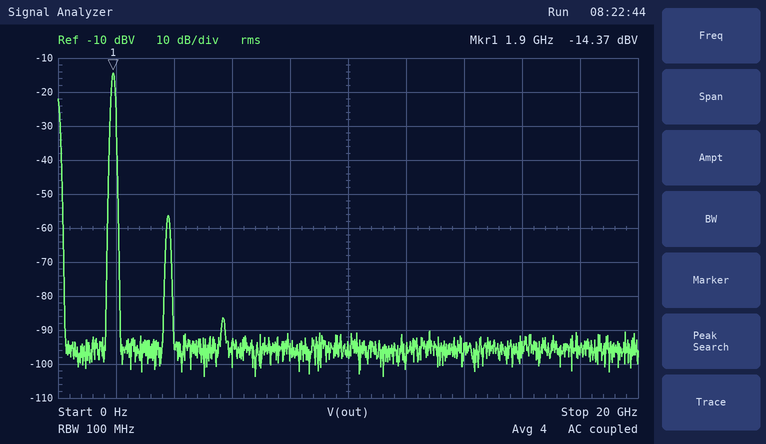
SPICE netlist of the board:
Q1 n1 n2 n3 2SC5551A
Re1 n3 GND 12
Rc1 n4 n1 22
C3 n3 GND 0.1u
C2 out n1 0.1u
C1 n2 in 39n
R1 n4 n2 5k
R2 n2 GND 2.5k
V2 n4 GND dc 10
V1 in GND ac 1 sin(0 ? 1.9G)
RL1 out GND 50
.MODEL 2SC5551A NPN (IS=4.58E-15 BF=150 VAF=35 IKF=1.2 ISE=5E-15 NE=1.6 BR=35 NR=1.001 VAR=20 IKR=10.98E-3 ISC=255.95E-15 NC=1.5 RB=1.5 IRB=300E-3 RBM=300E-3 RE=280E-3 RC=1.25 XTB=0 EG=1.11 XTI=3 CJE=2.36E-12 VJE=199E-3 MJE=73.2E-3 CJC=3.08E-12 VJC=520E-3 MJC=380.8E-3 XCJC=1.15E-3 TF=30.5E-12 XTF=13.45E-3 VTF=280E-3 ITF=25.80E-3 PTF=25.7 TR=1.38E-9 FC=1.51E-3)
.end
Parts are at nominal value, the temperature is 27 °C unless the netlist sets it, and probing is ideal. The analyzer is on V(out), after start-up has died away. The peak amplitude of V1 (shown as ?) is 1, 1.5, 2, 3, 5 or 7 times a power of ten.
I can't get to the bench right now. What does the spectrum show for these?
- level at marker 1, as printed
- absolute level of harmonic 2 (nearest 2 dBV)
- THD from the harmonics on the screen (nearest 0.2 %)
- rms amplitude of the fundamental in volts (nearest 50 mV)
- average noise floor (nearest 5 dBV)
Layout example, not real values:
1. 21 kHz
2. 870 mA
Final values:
1. -14.37 dBV
2. -56 dBV
3. 0.8 %
4. 200 mV
5. -95 dBV
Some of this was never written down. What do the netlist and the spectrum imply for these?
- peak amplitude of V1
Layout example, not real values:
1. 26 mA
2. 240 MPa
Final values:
1. 15 mV
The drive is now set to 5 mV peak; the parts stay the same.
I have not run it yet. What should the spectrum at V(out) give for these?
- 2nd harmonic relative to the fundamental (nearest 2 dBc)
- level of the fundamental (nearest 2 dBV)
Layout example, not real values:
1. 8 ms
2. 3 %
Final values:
1. -52 dBc
2. -24 dBV
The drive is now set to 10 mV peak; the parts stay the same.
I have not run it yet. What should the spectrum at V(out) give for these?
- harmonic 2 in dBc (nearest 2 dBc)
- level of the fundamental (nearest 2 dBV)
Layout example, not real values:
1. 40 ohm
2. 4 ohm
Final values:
1. -46 dBc
2. -18 dBV
